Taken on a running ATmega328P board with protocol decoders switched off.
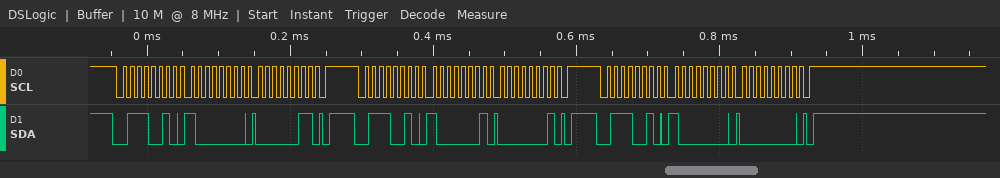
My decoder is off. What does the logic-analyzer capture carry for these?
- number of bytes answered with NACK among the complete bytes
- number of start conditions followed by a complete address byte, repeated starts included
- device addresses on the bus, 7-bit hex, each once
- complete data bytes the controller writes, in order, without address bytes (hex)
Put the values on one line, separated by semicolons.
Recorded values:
0; 3; 0x39; 80 03 81 01 80 00
